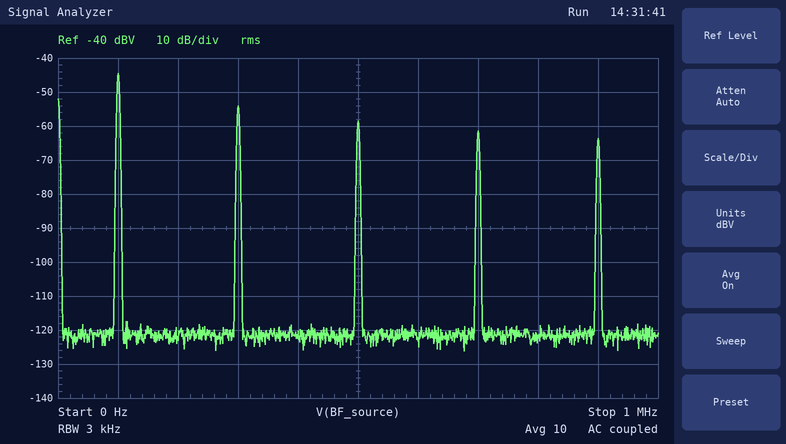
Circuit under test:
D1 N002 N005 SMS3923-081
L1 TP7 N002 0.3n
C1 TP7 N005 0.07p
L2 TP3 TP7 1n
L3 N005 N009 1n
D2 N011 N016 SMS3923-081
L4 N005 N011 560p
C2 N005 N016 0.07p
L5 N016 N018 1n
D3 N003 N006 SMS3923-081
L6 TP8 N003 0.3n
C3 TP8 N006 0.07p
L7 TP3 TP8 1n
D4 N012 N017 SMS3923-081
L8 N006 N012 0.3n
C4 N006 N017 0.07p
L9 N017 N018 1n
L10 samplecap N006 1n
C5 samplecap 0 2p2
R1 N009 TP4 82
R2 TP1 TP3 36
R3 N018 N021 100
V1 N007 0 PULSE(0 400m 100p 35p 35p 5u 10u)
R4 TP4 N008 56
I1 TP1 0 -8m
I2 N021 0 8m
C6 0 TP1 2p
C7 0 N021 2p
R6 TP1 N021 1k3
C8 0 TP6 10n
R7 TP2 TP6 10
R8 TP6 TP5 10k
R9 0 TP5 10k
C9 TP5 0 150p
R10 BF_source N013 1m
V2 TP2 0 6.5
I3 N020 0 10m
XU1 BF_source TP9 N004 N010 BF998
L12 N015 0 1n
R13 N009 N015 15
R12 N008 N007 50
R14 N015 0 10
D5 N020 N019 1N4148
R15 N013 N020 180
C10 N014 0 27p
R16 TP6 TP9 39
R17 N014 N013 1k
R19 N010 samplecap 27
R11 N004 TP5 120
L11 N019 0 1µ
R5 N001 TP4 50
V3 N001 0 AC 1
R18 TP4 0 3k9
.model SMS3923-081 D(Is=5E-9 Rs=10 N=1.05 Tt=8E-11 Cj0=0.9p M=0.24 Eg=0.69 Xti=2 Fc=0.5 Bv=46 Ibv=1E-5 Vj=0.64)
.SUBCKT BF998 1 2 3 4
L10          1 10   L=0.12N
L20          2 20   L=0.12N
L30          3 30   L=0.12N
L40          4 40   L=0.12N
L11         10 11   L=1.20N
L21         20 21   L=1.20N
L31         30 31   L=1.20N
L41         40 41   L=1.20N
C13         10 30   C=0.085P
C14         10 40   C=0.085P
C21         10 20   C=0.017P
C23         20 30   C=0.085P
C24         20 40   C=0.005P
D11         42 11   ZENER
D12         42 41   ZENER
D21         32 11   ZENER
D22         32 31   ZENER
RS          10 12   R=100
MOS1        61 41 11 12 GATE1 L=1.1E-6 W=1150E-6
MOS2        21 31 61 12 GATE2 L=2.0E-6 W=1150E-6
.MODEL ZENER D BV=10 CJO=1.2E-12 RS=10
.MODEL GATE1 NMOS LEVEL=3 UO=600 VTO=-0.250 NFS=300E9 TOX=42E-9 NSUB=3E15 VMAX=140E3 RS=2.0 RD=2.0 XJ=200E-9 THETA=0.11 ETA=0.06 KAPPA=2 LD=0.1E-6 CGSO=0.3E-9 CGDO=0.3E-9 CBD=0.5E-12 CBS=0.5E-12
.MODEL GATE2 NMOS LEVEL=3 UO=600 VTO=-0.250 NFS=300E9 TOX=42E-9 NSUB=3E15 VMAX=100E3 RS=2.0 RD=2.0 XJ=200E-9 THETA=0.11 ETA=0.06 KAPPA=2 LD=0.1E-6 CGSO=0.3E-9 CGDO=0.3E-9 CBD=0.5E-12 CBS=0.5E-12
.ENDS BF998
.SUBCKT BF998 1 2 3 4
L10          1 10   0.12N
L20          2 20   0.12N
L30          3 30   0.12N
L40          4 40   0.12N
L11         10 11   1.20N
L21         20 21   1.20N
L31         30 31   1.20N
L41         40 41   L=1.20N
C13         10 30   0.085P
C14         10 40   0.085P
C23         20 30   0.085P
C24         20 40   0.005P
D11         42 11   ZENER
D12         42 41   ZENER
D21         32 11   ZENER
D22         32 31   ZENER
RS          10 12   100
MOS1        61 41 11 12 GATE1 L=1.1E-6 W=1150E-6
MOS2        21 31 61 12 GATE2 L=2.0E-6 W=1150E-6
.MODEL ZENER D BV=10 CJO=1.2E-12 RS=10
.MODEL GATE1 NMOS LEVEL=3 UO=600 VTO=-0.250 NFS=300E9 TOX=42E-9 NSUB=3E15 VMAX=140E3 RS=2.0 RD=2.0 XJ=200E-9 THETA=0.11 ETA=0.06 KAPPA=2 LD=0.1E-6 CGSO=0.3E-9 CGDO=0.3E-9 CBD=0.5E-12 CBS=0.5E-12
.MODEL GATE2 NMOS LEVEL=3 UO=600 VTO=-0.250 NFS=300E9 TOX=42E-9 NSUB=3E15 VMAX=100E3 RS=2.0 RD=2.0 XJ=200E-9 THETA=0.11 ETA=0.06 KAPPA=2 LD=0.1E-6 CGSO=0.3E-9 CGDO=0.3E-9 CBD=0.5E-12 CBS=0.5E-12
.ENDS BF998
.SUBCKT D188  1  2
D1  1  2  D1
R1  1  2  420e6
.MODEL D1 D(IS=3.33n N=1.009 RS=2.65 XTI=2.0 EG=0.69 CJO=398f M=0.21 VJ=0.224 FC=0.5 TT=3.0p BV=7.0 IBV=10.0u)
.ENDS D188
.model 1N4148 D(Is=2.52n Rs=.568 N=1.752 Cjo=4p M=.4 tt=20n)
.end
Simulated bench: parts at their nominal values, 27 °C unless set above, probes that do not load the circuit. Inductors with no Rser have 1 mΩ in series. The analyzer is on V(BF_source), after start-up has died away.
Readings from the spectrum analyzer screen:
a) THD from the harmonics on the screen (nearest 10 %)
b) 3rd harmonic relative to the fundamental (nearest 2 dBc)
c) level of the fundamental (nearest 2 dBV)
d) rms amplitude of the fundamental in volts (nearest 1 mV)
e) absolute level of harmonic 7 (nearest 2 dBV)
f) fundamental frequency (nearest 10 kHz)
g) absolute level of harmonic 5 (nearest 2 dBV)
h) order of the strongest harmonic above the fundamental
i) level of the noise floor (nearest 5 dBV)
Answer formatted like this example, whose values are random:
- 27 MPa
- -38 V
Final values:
- 40 %
- -10 dBc
- -44 dBV
- 6 mV
- -62 dBV
- 100 kHz
- -58 dBV
- 3
- -120 dBV
